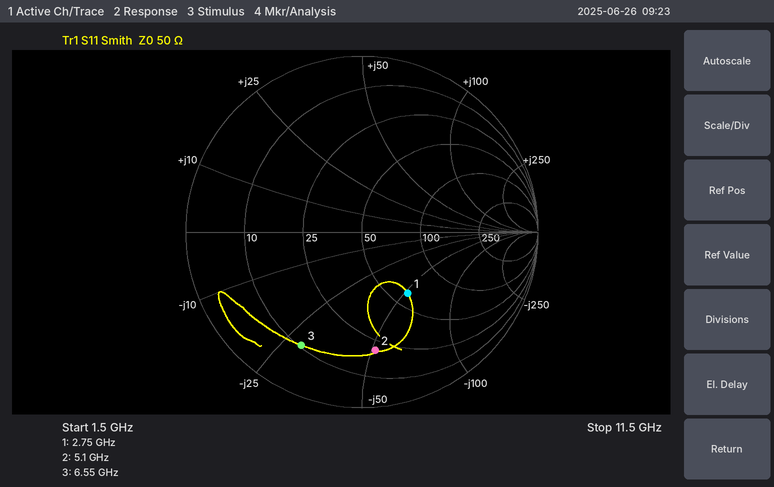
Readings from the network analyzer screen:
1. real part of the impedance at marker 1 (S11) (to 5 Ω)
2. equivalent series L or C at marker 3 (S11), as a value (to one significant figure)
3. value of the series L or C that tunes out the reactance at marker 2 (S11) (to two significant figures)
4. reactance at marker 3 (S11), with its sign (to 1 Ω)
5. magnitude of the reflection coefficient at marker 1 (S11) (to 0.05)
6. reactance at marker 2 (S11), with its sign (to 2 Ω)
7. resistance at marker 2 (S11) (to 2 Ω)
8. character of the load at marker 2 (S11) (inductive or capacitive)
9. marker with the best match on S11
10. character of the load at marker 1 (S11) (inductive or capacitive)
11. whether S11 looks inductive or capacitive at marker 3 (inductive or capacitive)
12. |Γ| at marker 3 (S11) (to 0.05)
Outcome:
60 Ω
800 fF
1.6 nH
-29 Ω
0.45
-52 Ω
20 Ω
capacitive
marker 1
capacitive
capacitive
0.75
